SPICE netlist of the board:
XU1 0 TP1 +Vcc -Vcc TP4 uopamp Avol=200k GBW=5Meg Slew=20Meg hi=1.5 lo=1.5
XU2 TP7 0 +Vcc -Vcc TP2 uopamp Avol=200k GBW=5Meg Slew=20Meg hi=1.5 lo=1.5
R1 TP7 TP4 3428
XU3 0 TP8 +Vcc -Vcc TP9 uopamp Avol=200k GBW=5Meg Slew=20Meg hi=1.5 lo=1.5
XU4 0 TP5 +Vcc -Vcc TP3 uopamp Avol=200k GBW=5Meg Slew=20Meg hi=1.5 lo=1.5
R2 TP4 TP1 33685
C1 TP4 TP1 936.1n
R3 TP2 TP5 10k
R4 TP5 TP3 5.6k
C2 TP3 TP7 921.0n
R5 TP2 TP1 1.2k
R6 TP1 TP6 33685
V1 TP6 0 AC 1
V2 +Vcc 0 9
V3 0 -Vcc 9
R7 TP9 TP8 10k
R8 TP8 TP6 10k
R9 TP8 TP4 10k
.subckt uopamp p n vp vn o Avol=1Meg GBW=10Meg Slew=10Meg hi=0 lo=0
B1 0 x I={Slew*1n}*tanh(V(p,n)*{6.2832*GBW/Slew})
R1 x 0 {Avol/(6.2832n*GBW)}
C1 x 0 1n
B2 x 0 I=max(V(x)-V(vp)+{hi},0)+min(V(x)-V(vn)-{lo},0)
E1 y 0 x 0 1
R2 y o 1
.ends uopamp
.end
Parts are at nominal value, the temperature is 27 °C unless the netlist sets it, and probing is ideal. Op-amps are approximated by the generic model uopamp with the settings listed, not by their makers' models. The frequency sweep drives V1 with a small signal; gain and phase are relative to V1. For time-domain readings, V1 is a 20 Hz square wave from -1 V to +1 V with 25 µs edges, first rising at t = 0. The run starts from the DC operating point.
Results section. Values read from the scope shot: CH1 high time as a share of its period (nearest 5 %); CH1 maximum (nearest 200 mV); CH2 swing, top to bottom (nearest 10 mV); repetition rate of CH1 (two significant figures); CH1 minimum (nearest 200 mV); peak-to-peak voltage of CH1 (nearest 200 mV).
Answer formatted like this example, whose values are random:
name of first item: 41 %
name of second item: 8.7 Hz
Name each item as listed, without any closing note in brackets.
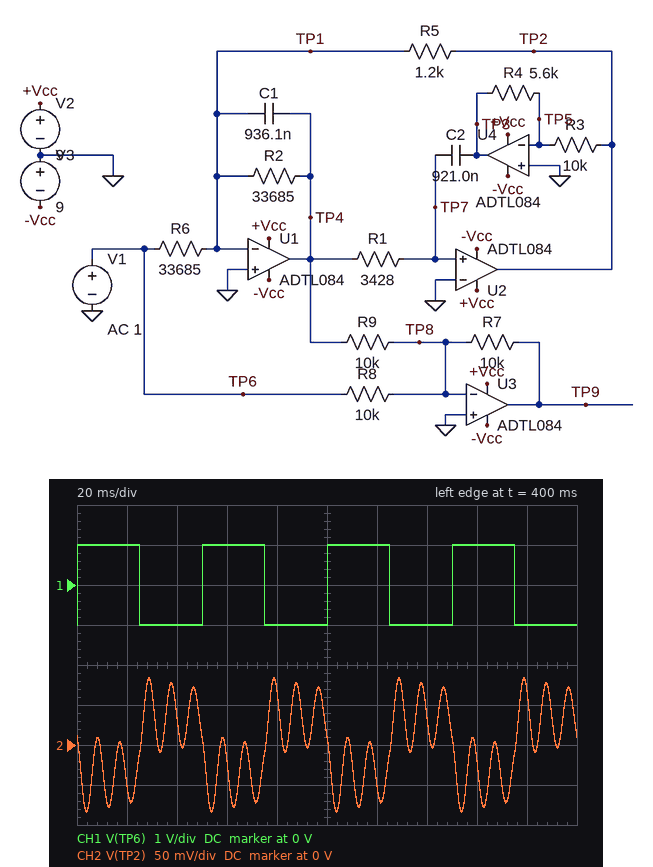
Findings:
CH1 high time as a share of its period: 50 %
CH1 maximum: 1.0 V
CH2 swing, top to bottom: 170 mV
repetition rate of CH1: 20 Hz
CH1 minimum: -1.0 V
peak-to-peak voltage of CH1: 2.0 V
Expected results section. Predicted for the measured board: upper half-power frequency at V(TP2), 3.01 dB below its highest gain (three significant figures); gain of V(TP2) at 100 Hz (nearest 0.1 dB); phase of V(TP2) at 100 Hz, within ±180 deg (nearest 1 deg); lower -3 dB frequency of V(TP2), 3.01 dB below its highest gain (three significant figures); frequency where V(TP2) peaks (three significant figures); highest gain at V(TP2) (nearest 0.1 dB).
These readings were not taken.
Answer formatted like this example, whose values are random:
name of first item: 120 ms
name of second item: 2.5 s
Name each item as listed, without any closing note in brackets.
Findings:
upper half-power frequency at V(TP2), 3.01 dB below its highest gain: 115 Hz
gain of V(TP2) at 100 Hz: -15.8 dB
phase of V(TP2) at 100 Hz, within ±180 deg: 170 deg
lower -3 dB frequency of V(TP2), 3.01 dB below its highest gain: 110 Hz
frequency where V(TP2) peaks: 113 Hz
highest gain at V(TP2): -2.0 dB
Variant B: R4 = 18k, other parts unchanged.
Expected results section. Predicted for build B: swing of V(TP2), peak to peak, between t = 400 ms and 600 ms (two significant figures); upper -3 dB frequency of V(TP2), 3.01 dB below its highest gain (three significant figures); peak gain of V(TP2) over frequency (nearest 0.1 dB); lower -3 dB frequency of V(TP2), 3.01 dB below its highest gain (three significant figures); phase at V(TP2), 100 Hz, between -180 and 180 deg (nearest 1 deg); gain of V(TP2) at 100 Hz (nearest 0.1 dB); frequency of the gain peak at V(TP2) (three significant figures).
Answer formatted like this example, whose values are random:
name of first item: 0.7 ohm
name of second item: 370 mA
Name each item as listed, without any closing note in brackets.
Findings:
swing of V(TP2), peak to peak, between t = 400 ms and 600 ms: 330 mV
upper -3 dB frequency of V(TP2), 3.01 dB below its highest gain: 65.4 Hz
peak gain of V(TP2) over frequency: -7.0 dB
lower -3 dB frequency of V(TP2), 3.01 dB below its highest gain: 60.3 Hz
phase at V(TP2), 100 Hz, between -180 and 180 deg: 5 deg
gain of V(TP2) at 100 Hz: -32.6 dB
frequency of the gain peak at V(TP2): 62.9 Hz
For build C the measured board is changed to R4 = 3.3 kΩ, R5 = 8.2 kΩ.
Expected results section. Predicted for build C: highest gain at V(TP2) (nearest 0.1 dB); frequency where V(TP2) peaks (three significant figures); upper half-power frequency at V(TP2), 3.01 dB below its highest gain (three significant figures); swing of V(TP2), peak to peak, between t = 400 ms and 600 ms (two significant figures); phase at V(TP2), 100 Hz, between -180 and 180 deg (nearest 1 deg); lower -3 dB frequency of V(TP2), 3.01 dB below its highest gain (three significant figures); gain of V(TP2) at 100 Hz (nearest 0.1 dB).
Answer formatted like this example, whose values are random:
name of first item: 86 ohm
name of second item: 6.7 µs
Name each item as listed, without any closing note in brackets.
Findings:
highest gain at V(TP2): 8.7 dB
frequency where V(TP2) peaks: 56.2 Hz
upper half-power frequency at V(TP2), 3.01 dB below its highest gain: 58.6 Hz
swing of V(TP2), peak to peak, between t = 400 ms and 600 ms: 1.9 V
phase at V(TP2), 100 Hz, between -180 and 180 deg: 4 deg
lower -3 dB frequency of V(TP2), 3.01 dB below its highest gain: 53.6 Hz
gain of V(TP2) at 100 Hz: -19.0 dB
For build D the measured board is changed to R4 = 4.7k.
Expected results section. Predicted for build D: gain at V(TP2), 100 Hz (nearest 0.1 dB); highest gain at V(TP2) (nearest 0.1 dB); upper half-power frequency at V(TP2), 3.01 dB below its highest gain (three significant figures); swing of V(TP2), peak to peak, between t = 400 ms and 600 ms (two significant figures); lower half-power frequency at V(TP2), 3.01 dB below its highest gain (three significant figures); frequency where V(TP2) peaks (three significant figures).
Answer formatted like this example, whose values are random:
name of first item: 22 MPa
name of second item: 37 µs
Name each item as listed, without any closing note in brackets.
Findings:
gain at V(TP2), 100 Hz: -19.7 dB
highest gain at V(TP2): -1.2 dB
upper half-power frequency at V(TP2), 3.01 dB below its highest gain: 126 Hz
swing of V(TP2), peak to peak, between t = 400 ms and 600 ms: 150 mV
lower half-power frequency at V(TP2), 3.01 dB below its highest gain: 121 Hz
frequency where V(TP2) peaks: 123 Hz
